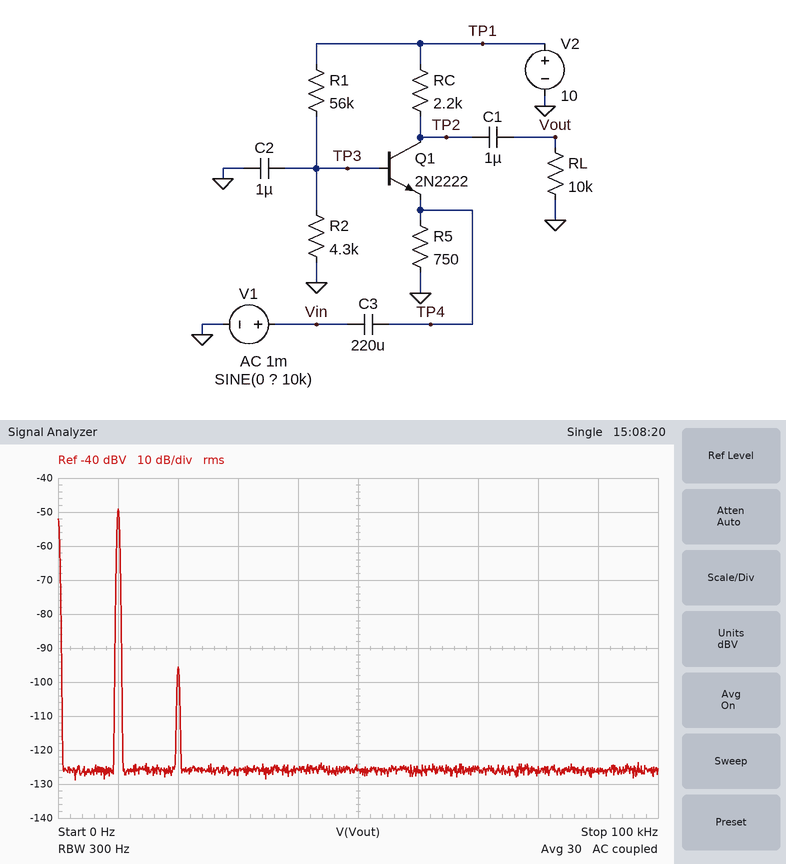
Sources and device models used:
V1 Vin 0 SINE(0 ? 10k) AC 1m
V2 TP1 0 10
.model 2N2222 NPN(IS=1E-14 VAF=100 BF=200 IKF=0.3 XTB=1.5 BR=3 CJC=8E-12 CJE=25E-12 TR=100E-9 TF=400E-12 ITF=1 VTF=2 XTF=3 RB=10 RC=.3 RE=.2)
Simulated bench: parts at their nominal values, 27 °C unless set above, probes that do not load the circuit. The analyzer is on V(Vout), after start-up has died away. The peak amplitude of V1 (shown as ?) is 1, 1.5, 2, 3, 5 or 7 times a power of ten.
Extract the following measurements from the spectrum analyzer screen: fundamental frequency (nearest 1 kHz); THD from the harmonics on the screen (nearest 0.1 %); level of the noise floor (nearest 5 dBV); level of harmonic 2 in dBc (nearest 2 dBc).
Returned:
10 kHz
0.5 %
-125 dBV
-46 dBc
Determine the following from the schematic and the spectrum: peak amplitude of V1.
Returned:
500 µV
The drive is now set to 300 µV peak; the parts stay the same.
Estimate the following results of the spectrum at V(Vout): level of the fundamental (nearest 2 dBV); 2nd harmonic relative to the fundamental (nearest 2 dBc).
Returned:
-54 dBV
-50 dBc
